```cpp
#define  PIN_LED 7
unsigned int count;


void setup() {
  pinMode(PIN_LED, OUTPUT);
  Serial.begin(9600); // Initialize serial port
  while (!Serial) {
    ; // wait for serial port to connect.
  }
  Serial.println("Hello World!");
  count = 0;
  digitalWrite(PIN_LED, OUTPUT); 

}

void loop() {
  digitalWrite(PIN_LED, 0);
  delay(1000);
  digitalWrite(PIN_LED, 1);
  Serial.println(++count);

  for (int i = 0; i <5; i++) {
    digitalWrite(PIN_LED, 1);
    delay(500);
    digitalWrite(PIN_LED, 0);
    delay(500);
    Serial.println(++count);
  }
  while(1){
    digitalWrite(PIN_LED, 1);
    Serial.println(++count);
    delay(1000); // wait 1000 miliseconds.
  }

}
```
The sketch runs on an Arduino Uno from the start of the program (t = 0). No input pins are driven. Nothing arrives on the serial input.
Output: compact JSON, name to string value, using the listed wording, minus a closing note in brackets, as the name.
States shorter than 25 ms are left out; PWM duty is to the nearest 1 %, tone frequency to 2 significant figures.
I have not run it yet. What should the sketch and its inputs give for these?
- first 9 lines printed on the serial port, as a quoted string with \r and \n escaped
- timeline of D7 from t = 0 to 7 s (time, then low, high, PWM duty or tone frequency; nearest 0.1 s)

{"first 9 lines printed on the serial port, as a quoted string with \\r and \\n escaped": "\"Hello World!\\r\\n1\\r\\n2\\r\\n3\\r\\n4\\r\\n5\\r\\n6\\r\\n7\\r\\n8\\r\\n\"", "timeline of D7 from t = 0 to 7 s": "0 s low; 1 s high; 1.5 s low; 2 s high; 2.5 s low; 3 s high; 3.5 s low; 4 s high; 4.5 s low; 5 s high; 5.5 s low; 6 s high"}
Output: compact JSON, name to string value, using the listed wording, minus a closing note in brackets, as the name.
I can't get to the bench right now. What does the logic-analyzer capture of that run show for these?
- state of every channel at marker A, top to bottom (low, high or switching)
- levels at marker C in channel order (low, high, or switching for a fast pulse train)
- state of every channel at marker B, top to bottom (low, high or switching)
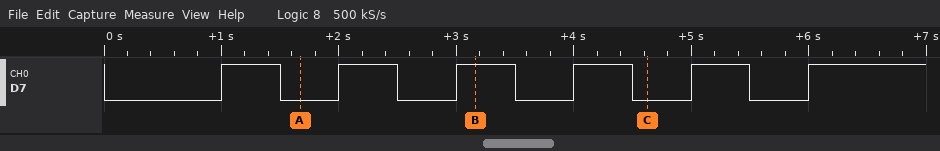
{"state of every channel at marker A, top to bottom": "D7 low", "levels at marker C in channel order": "D7 low", "state of every channel at marker B, top to bottom": "D7 high"}
